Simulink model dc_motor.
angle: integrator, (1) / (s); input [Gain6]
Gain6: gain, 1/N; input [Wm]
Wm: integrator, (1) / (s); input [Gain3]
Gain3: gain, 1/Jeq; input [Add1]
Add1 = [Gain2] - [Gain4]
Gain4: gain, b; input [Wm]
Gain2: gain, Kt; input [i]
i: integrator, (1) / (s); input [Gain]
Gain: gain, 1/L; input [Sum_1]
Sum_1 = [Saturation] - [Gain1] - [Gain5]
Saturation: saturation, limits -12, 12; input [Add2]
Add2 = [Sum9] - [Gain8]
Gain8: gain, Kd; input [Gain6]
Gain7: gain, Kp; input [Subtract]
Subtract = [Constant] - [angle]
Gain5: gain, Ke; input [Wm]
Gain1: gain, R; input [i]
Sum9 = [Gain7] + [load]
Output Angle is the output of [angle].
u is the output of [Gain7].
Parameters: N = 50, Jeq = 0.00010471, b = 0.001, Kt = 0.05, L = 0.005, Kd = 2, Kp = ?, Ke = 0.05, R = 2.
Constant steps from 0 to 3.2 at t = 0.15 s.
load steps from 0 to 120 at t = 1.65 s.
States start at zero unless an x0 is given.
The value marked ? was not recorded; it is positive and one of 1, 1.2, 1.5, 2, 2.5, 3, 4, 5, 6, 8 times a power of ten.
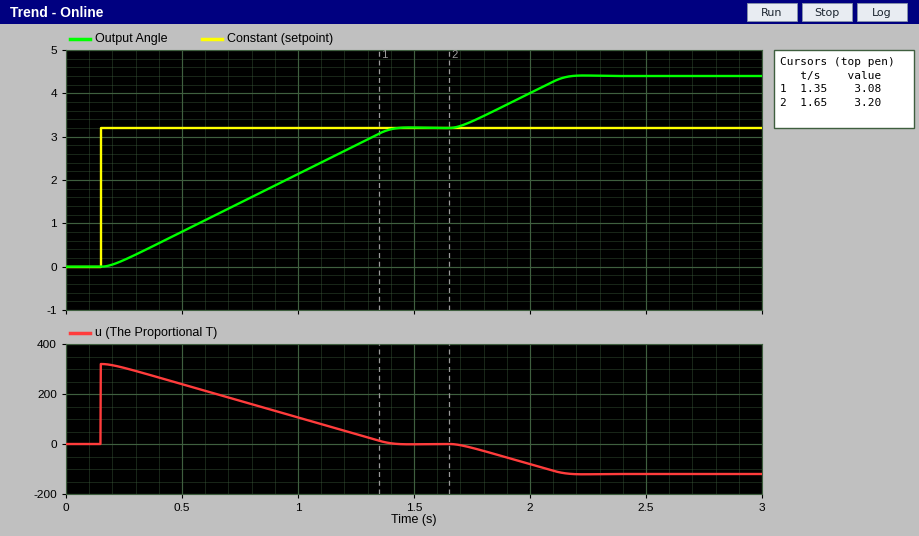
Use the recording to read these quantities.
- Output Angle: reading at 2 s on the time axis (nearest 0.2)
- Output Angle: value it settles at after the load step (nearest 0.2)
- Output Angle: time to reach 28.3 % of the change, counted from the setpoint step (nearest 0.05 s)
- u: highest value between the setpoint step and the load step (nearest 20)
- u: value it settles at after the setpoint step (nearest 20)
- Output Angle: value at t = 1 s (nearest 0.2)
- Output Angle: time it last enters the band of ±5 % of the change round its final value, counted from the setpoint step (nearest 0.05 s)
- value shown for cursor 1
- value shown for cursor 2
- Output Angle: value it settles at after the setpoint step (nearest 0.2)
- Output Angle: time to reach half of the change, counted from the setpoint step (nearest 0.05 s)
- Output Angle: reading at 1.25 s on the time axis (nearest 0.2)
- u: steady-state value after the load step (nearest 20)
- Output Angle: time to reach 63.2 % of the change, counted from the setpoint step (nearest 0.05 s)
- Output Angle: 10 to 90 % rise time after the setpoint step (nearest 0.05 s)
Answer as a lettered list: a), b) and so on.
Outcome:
a) 4.0
b) 4.4
c) 0.40 s
d) 320
e) 0
f) 2.2
g) 1.20 s
h) 3.08
i) 3.20
j) 3.2
k) 0.65 s
l) 2.8
m) -120
n) 0.80 s
o) 0.95 s
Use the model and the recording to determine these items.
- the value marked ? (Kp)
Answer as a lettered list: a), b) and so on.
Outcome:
a) 100
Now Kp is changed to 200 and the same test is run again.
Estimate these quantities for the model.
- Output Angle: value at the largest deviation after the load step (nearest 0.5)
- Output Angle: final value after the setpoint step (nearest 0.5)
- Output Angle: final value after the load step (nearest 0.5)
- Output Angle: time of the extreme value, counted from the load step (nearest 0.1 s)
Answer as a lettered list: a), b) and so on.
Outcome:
a) 4.0
b) 3.0
c) 4.0
d) 0.3 s
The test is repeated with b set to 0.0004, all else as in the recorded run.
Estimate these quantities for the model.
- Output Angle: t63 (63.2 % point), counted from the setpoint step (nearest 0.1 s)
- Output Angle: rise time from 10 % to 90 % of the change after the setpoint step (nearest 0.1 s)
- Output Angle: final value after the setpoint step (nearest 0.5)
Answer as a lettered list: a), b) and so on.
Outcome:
a) 0.6 s
b) 0.7 s
c) 3.0
